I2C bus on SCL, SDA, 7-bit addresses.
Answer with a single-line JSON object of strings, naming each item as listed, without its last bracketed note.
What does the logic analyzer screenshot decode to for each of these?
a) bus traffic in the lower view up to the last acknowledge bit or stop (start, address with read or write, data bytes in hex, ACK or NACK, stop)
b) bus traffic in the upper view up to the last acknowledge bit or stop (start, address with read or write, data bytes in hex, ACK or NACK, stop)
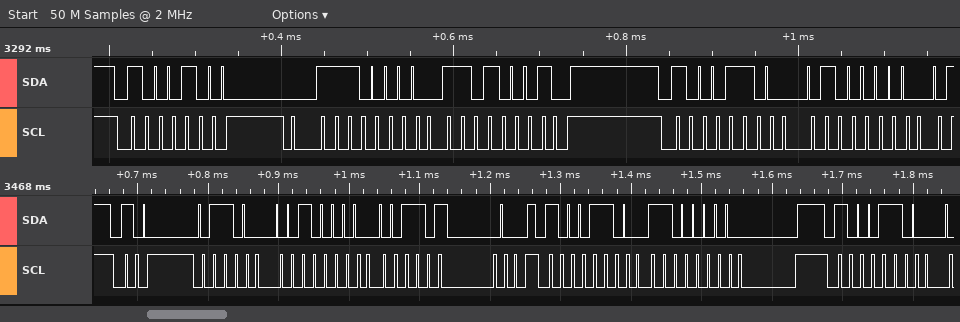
{"bus traffic in the lower view up to the last acknowledge bit or stop": "start, address 46 write ACK, 20 ACK, 34 ACK, stop, start, address 46 write ACK, C0 ACK, stop, start, address 46 write ACK", "bus traffic in the upper view up to the last acknowledge bit or stop": "start, address 44 write ACK, E0 ACK, D1 ACK, stop, start, address 46 write ACK, 40 ACK"}
